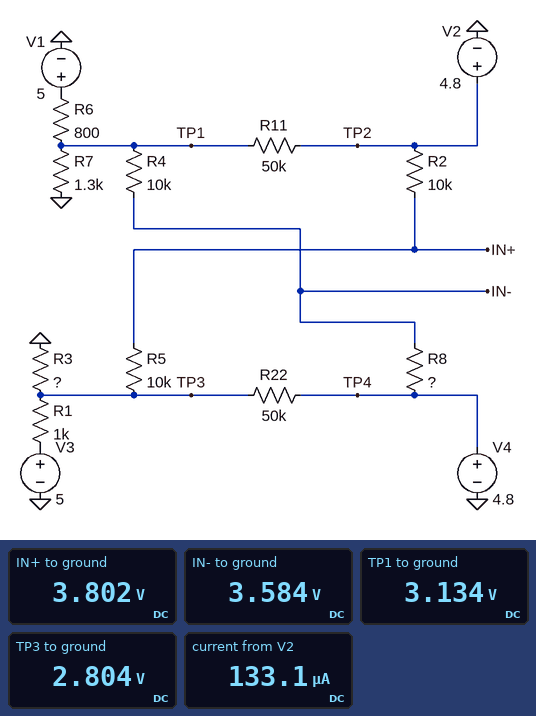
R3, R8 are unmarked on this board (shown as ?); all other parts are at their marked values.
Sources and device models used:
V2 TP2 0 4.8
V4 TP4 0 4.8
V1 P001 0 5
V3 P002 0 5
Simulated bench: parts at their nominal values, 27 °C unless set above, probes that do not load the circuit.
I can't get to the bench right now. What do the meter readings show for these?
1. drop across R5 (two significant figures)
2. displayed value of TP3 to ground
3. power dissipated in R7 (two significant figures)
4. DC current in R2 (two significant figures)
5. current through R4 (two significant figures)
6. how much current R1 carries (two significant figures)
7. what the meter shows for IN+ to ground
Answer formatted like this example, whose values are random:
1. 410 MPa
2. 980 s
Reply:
1. 1.0 V
2. 2.804 V
3. 7.6 mW
4. 100 µA
5. 45 µA
6. 2.2 mA
7. 3.802 V
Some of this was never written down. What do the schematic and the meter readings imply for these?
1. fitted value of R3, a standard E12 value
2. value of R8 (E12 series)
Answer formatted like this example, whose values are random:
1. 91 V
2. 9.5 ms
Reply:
1. 1.2 kΩ
2. 27 kΩ
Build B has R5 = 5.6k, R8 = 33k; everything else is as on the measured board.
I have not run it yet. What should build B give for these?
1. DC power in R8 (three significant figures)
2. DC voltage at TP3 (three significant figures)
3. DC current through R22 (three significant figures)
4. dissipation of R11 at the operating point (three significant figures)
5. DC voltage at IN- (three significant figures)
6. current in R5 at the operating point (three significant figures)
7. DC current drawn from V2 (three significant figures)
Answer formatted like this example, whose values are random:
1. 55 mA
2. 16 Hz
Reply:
1. 49.7 µW
2. 2.82 V
3. 39.6 µA
4. 55.7 µW
5. 3.52 V
6. 127 µA
7. 160 µA
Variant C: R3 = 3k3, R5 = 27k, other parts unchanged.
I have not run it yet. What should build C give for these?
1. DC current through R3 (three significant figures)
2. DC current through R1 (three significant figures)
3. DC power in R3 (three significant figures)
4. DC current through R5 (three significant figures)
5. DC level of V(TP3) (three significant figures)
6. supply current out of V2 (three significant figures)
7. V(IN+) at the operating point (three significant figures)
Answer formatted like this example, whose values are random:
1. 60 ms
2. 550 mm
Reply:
1. 1.17 mA
2. 1.13 mA
3. 4.54 mW
4. 25.1 µA
5. 3.87 V
6. 58.4 µA
7. 4.55 V
